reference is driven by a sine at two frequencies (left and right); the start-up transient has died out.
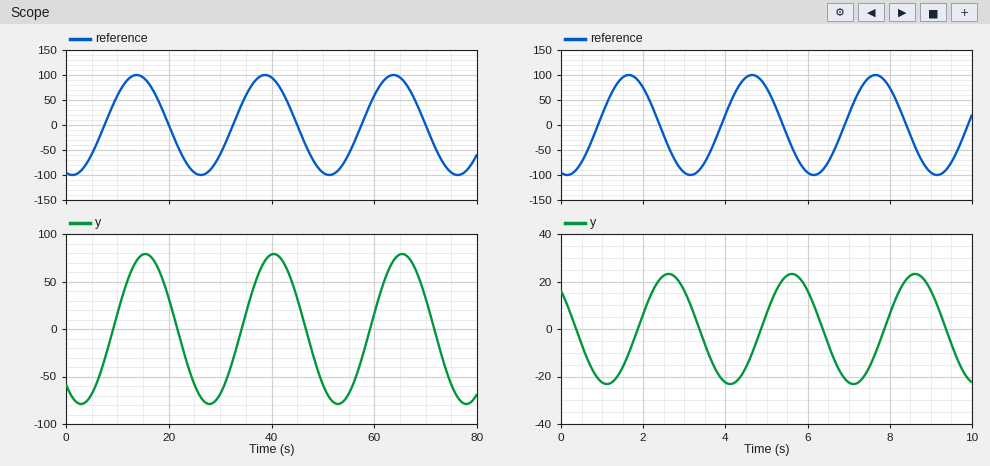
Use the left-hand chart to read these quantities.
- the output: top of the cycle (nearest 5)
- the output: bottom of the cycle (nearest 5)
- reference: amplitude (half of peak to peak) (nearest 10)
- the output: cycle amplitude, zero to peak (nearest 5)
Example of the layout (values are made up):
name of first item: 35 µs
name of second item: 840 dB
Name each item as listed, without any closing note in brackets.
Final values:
the output: top of the cycle: 80
the output: bottom of the cycle: -80
reference: amplitude (half of peak to peak): 100
the output: cycle amplitude, zero to peak: 80
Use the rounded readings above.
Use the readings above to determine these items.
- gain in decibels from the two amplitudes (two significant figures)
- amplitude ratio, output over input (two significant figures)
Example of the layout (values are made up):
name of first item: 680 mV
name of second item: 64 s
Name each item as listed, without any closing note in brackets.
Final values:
gain in decibels from the two amplitudes: -1.9 dB
amplitude ratio, output over input: 0.80
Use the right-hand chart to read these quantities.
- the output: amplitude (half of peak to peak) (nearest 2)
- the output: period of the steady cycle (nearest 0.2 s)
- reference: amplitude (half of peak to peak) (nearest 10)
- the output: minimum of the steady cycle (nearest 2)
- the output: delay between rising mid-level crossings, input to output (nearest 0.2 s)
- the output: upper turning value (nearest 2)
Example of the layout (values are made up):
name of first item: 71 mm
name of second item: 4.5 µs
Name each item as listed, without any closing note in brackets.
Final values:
the output: amplitude (half of peak to peak): 24
the output: period of the steady cycle: 3.0 s
reference: amplitude (half of peak to peak): 100
the output: minimum of the steady cycle: -24
the output: delay between rising mid-level crossings, input to output: 1.0 s
the output: upper turning value: 24
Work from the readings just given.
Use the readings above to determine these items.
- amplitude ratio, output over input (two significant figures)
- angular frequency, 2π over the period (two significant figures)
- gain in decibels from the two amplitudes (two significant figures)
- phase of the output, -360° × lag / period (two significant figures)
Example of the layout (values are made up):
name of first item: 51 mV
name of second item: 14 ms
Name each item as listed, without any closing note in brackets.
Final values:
amplitude ratio, output over input: 0.24
angular frequency, 2π over the period: 2.1 rad/s
gain in decibels from the two amplitudes: -12 dB
phase of the output, -360° × lag / period: -120°
